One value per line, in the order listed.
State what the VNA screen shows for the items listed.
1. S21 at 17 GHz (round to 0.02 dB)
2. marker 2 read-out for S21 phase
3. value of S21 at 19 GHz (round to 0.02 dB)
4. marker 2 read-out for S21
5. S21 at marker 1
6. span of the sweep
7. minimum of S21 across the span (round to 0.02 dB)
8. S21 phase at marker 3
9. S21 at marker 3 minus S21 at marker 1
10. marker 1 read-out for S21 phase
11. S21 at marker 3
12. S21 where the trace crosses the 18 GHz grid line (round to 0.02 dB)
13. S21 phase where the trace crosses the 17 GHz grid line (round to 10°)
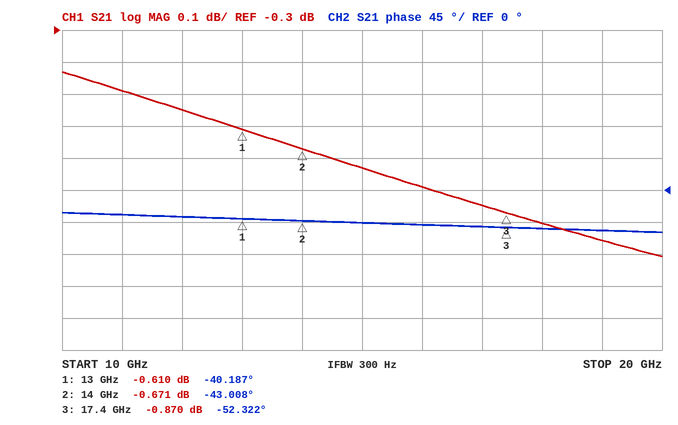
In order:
-0.84 dB
-43.008°
-0.96 dB
-0.671 dB
-0.610 dB
10 GHz
-1.00 dB
-52.322°
-0.260 dB
-40.187°
-0.870 dB
-0.90 dB
-50°
